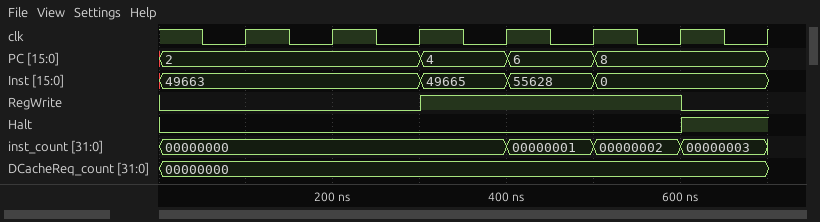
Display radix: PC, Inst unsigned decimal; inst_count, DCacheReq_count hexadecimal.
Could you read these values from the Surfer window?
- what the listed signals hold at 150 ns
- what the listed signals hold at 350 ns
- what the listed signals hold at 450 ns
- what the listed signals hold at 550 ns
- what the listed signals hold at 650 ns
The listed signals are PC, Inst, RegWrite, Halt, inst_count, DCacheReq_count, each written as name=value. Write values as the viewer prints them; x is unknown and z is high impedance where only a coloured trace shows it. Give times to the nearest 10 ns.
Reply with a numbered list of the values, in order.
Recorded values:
1. PC=2, Inst=49663, RegWrite=0, Halt=0, inst_count=00000000, DCacheReq_count=00000000
2. PC=4, Inst=49665, RegWrite=1, Halt=0, inst_count=00000000, DCacheReq_count=00000000
3. PC=6, Inst=55628, RegWrite=1, Halt=0, inst_count=00000001, DCacheReq_count=00000000
4. PC=8, Inst=0, RegWrite=1, Halt=0, inst_count=00000002, DCacheReq_count=00000000
5. PC=8, Inst=0, RegWrite=0, Halt=1, inst_count=00000003, DCacheReq_count=00000000
